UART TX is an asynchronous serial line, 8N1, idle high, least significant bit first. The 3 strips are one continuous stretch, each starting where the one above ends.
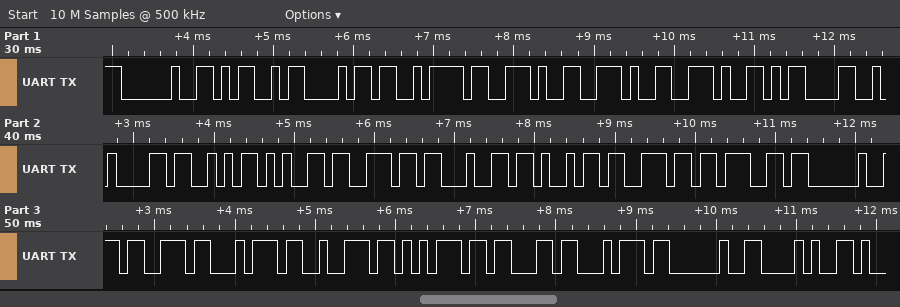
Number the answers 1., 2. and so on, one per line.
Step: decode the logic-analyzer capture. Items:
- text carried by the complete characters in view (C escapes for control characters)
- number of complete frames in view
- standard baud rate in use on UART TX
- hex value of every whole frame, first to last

1. " Mhz...\r\nSending struct ("
2. 25
3. 9600 baud
4. 0x20 0x4D 0x68 0x7A 0x2E 0x2E 0x2E 0x0D 0x0A 0x53 0x65 0x6E 0x64 0x69 0x6E 0x67 0x20 0x73 0x74 0x72 0x75 0x63 0x74 0x20 0x28
